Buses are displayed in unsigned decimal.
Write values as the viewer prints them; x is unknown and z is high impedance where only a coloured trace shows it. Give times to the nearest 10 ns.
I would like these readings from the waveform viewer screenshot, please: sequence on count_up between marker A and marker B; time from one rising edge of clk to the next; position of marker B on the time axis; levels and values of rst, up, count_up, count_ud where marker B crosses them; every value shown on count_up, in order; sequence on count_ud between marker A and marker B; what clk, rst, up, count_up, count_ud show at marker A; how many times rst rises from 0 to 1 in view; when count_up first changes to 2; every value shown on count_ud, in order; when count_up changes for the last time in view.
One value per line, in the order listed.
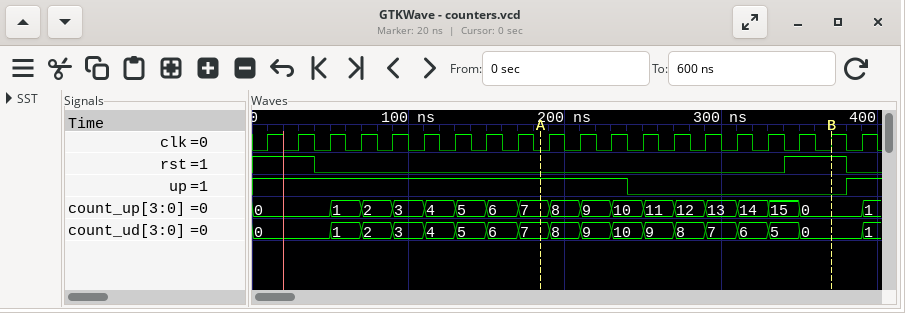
7, 8, 9, 10, 11, 12, 13, 14, 15, 0
20 ns
370 ns
rst=1, up=0, count_up=0, count_ud=0
0, 1, 2, 3, 4, 5, 6, 7, 8, 9, 10, 11, 12, 13, 14, 15, 0, 1
7, 8, 9, 10, 9, 8, 7, 6, 5, 0
clk=0, rst=0, up=1, count_up=7, count_ud=7
1
70 ns
0, 1, 2, 3, 4, 5, 6, 7, 8, 9, 10, 9, 8, 7, 6, 5, 0, 1
390 ns
